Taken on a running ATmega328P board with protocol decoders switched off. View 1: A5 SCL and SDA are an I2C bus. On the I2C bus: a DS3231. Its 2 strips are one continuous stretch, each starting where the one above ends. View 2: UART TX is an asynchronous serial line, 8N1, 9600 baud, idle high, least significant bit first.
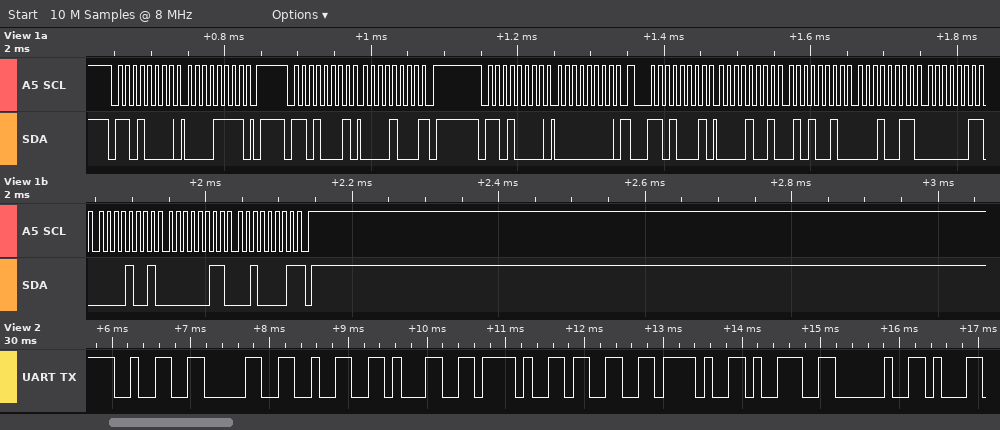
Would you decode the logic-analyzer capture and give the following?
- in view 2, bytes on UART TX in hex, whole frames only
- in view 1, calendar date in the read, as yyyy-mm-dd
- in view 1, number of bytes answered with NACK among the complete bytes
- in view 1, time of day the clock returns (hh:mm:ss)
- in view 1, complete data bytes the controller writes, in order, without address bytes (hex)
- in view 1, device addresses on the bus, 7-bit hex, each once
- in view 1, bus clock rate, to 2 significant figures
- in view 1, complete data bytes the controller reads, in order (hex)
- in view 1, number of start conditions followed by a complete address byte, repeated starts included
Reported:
32 30 32 31 2F 33 2F 39 20
2021-03-09
2
13:52:09
0F 00
0x68
100 kHz
08 09 52 13 03 09 03 21
4
